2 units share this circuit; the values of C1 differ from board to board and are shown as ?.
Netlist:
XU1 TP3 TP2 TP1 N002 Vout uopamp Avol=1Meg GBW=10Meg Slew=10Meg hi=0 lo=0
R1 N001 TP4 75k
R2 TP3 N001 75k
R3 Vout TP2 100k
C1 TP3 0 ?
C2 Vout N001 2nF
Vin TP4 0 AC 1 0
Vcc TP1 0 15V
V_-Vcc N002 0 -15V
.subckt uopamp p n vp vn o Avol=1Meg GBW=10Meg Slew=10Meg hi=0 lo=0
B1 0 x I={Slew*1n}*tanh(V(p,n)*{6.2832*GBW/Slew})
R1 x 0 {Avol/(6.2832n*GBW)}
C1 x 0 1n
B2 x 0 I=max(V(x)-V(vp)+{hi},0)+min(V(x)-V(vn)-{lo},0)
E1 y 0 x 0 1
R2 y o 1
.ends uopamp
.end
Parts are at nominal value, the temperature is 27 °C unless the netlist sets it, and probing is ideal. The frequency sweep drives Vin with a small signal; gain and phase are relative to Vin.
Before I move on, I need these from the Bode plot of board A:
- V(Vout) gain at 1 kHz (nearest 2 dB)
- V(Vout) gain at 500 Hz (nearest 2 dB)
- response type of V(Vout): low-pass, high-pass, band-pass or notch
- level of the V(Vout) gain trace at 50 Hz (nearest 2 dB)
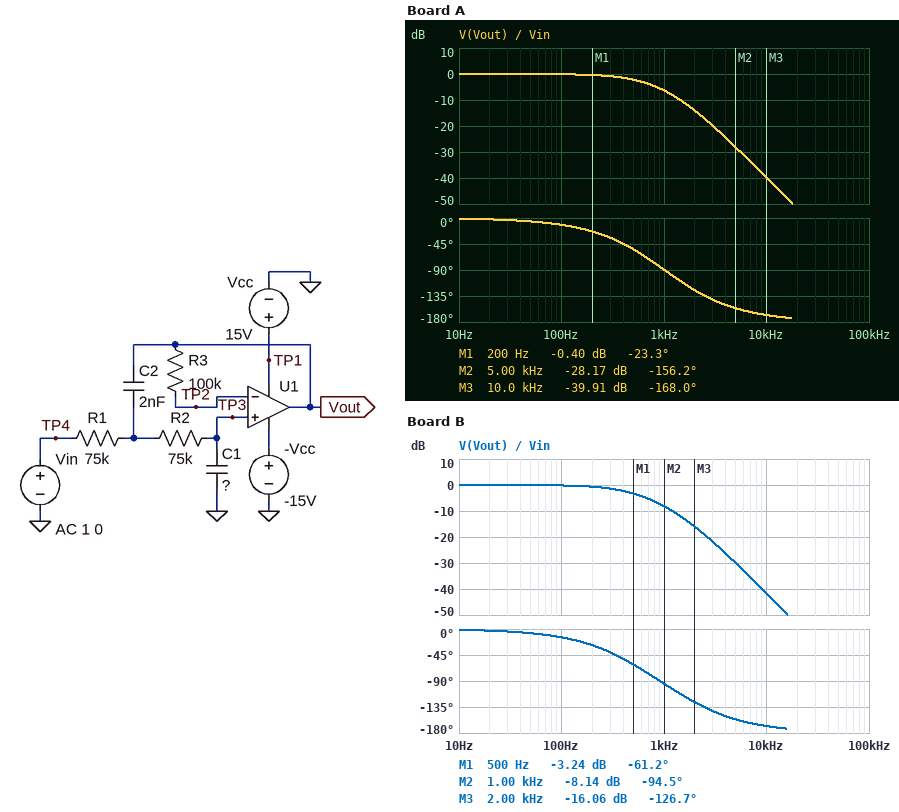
-6 dB
-2 dB
low-pass
0 dB
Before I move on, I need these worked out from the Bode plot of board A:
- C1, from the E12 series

2.2 nF
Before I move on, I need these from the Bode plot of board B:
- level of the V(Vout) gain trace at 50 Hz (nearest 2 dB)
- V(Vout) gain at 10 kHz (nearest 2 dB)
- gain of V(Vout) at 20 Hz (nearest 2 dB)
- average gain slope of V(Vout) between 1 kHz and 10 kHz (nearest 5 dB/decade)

0 dB
-42 dB
0 dB
-35 dB/decade
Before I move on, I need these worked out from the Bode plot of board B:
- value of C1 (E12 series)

2.7 nF
